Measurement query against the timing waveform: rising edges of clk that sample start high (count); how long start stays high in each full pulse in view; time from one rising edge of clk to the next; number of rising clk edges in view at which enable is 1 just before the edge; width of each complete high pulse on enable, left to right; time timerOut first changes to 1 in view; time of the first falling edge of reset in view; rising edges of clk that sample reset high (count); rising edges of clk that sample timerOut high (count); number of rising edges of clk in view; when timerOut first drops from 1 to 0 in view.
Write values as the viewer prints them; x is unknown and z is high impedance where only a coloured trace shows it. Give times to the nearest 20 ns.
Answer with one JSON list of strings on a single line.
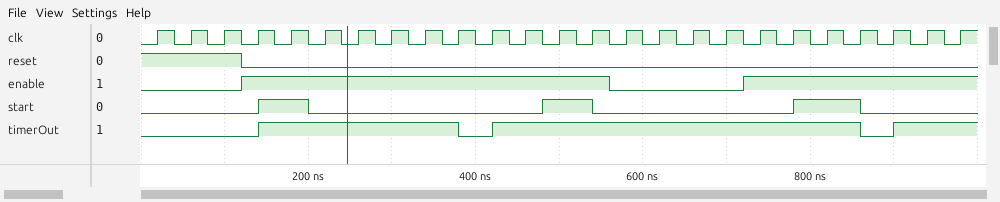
["5", "60 ns, 60 ns, 80 ns", "40 ns", "18", "440 ns", "140 ns", "120 ns", "3", "19", "25", "380 ns"]
